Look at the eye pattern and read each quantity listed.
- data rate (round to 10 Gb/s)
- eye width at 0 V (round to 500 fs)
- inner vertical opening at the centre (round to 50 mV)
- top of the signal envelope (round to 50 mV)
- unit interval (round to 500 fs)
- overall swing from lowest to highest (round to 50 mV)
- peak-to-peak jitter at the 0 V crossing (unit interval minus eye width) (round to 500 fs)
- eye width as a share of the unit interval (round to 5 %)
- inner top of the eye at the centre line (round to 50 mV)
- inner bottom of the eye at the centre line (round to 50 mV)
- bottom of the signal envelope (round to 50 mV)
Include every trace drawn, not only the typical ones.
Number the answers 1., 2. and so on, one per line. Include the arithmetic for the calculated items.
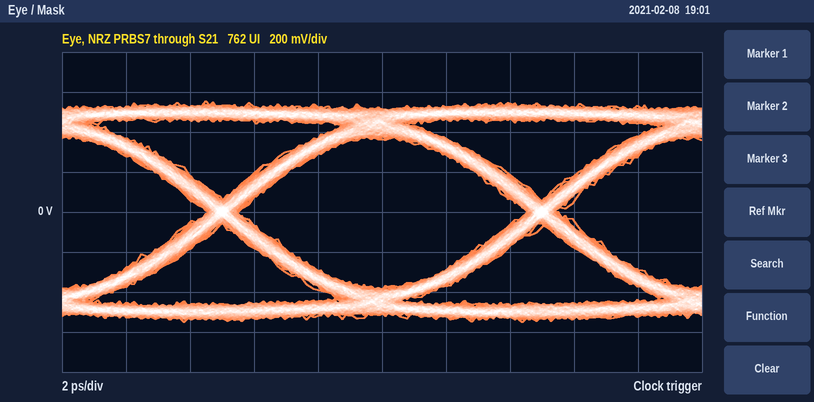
1. 100 Gb/s
2. 9.0 ps
3. 750 mV
4. 550 mV
5. 10.0 ps
6. 1.10 V
7. 1.0 ps
8. 9.0 ps / 10.0 ps ≈ 90 %
9. 350 mV
10. -400 mV
11. -550 mV
